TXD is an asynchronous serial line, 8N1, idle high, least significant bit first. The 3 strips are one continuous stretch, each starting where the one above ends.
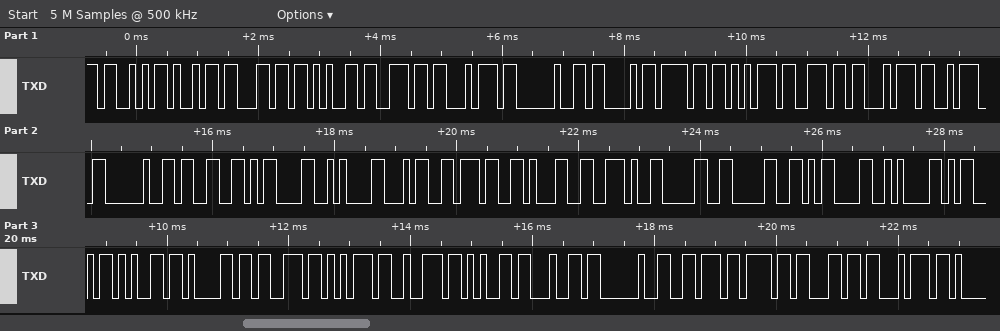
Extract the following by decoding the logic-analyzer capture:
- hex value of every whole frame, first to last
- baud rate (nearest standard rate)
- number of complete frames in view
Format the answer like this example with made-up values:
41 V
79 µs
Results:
0x53 0x69 0x6C 0x65 0x6E 0x74 0x20 0x43 0x6F 0x75 0x6E 0x74 0x3A 0x20 0x33 0x0D 0x0A 0x34 0x37 0x31 0x2E 0x30 0x30 0x0D 0x0A 0x4D 0x65 0x61 0x73 0x75 0x72 0x65 0x64 0x20 0x76 0x6F 0x6C 0x74
9600 baud
38
